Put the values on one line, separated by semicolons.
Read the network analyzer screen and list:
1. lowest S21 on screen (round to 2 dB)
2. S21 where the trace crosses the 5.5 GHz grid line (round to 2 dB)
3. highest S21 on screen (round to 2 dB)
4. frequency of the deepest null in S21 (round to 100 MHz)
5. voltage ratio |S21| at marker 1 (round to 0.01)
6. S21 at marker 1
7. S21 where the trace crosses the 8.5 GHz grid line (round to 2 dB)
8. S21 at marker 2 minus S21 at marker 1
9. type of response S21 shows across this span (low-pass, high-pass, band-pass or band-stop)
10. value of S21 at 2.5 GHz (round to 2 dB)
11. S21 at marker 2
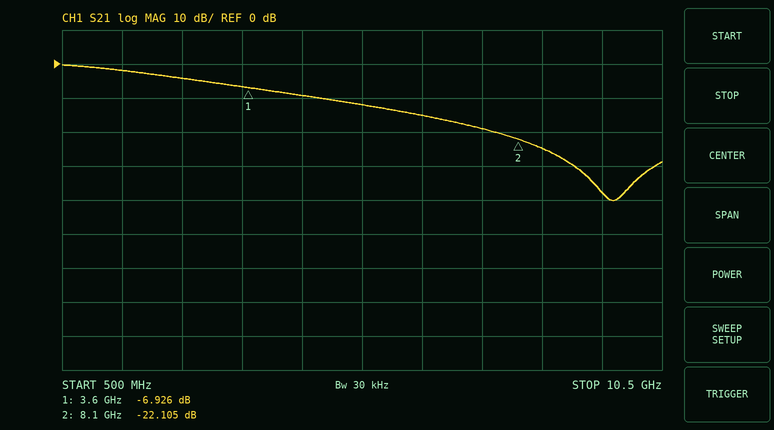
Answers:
-40 dB; -12 dB; 0 dB; 9.7 GHz; 0.45; -6.926 dB; -24 dB; -15.179 dB; low-pass; -4 dB; -22.105 dB
